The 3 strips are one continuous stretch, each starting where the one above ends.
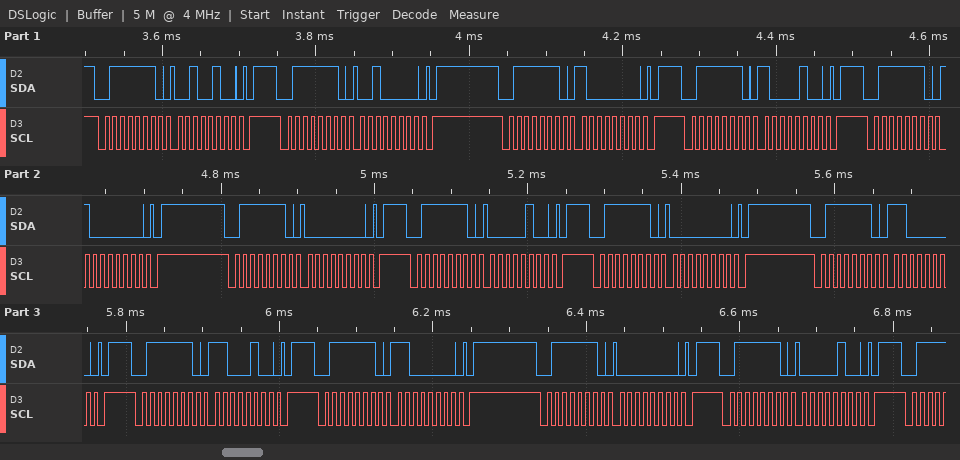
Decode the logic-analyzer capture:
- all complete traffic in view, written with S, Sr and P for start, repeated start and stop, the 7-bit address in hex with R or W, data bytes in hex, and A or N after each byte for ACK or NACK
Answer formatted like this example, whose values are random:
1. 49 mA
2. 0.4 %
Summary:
1. S 3FW A 24 A P S 3FW A 20 A P S 3FW A 80 A P S 3FW A 84 A P S 3FW A 80 A P S 3FW A 00 A P S 3FW A 04 A P S 3FW A 00 A P S 3FW A C0 A P S 3FW A C4 A P S 3FW A C0 A P S 3FW A 00 A P S 3FW A 04 A P
